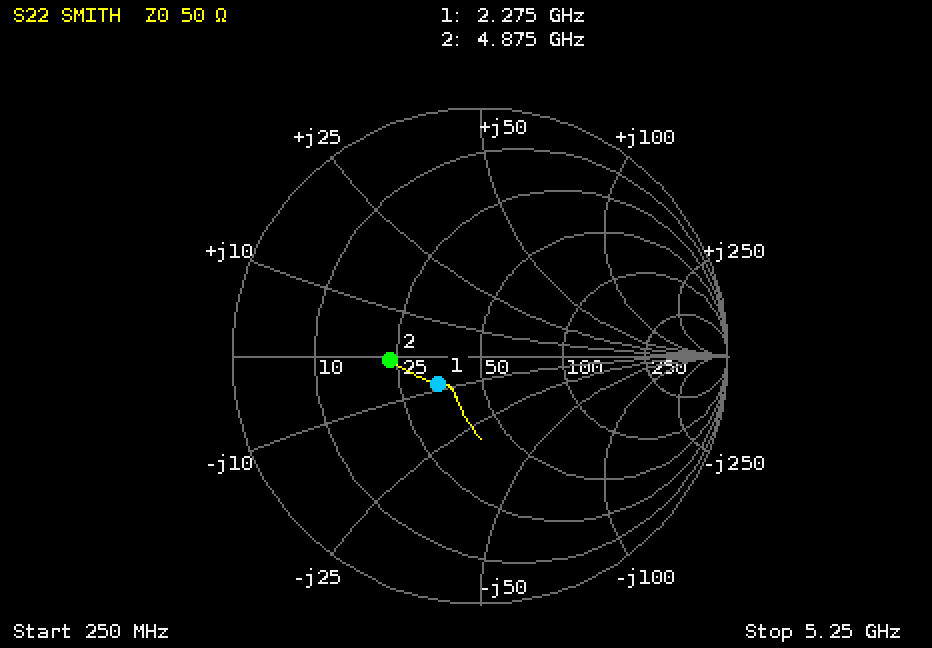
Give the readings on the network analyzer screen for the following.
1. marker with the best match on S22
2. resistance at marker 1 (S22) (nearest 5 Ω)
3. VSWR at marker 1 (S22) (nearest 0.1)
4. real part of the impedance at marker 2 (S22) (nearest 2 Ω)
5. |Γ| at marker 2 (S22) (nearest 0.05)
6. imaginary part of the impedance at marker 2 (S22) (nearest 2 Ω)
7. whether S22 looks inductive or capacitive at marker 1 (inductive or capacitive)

marker 1
35 Ω
1.5
24 Ω
0.35
0 Ω
capacitive
